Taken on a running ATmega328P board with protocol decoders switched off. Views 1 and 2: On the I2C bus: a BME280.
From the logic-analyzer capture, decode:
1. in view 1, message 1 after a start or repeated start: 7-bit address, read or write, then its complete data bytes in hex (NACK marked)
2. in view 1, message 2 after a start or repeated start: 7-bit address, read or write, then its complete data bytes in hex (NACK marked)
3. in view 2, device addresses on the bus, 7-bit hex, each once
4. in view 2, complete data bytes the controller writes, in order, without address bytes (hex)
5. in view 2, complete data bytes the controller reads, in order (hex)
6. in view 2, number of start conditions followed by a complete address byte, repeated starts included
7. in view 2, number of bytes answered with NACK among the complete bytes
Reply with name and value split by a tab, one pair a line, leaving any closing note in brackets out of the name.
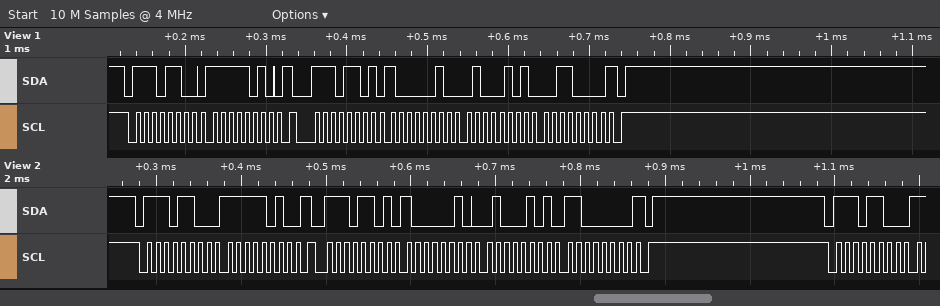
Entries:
in view 1, message 1 after a start or repeated start: 7-bit address, read or write, then its complete data bytes in hex	0x76 write: FA
in view 1, message 2 after a start or repeated start: 7-bit address, read or write, then its complete data bytes in hex	0x76 read: 82 45 30 NACK
in view 2, device addresses on the bus, 7-bit hex, each once	0x76
in view 2, complete data bytes the controller writes, in order, without address bytes	FA
in view 2, complete data bytes the controller reads, in order	82 45 C0
in view 2, number of start conditions followed by a complete address byte, repeated starts included	3
in view 2, number of bytes answered with NACK among the complete bytes	1
